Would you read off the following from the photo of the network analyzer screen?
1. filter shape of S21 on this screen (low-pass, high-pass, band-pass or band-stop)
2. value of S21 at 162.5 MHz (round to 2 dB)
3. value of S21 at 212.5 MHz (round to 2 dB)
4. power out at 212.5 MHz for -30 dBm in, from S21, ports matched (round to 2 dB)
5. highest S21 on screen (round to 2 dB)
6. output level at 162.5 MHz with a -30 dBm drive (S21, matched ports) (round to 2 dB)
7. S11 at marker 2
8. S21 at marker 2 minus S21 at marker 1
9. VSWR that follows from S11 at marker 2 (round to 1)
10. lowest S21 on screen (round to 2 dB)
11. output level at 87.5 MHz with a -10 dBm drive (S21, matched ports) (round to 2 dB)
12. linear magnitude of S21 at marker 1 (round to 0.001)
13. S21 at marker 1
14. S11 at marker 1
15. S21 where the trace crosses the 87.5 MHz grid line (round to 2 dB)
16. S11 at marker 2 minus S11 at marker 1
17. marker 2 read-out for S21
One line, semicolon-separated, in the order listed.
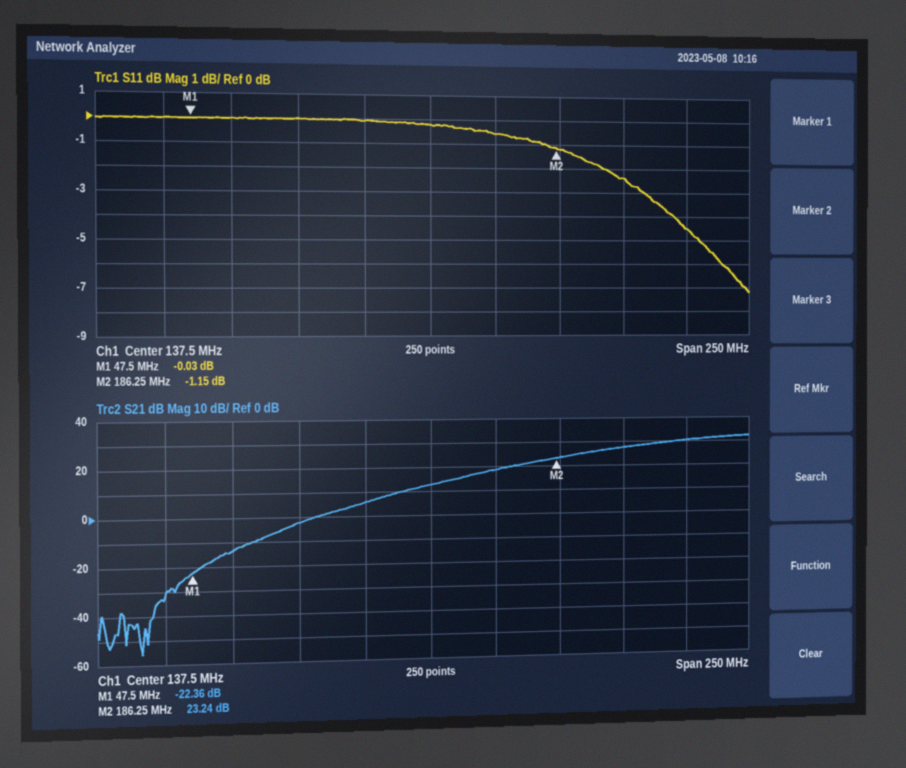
high-pass; 18 dB; 28 dB; -2 dBm; 32 dB; -12 dBm; -1.15 dB; 45.60 dB; 15; -56 dB; -12 dBm; 0.076; -22.36 dB; -0.03 dB; -2 dB; -1.12 dB; 23.24 dB
